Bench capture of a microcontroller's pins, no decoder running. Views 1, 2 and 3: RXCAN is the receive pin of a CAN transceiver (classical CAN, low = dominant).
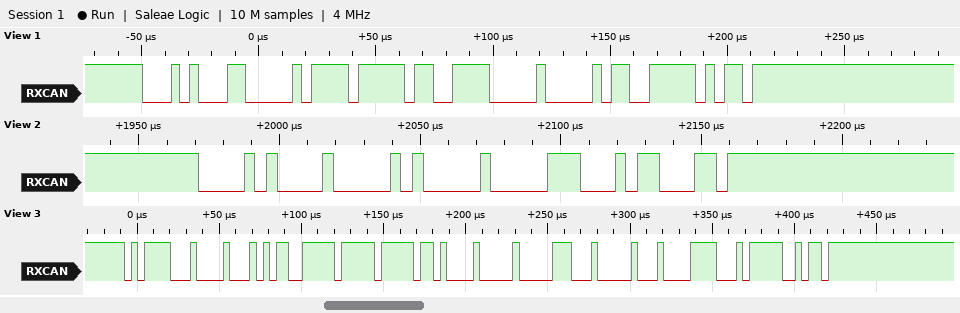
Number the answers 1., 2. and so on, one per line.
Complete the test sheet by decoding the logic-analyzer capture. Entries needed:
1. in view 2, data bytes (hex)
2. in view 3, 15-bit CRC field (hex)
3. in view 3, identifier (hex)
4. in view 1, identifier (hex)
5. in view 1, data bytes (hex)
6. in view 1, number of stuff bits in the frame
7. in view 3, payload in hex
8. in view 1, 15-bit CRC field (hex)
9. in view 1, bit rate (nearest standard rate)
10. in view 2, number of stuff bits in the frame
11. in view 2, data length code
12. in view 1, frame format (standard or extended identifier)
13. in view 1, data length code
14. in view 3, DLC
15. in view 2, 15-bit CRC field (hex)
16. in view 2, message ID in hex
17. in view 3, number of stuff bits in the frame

1. 00
2. 0x45F5
3. 0x5E2
4. 0x146
5. DF CF 00
6. 5
7. AC FF FF A1 00 31 00 87
8. 0x0CFD
9. 250 kbit/s
10. 3
11. 1
12. standard
13. 3
14. 8
15. 0x18B1
16. 0x0A1
17. 7
